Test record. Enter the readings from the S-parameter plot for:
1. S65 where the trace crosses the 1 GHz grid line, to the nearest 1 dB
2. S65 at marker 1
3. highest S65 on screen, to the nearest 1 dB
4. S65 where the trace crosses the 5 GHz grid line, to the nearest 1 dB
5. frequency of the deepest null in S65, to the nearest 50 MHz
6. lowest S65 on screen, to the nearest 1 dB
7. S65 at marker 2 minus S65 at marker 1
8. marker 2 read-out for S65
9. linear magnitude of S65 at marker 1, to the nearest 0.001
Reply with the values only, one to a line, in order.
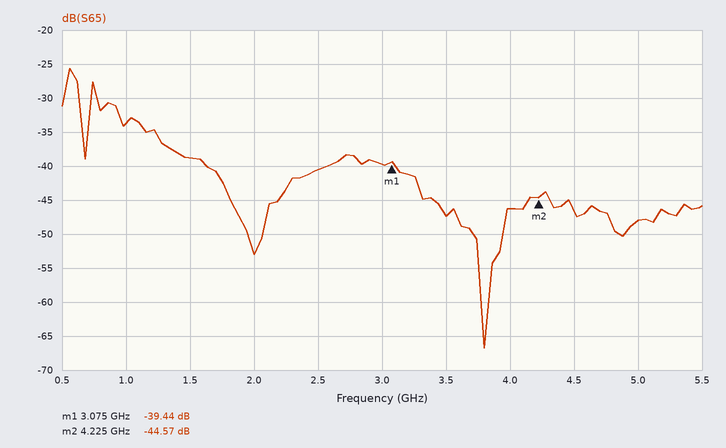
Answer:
-34 dB
-39.44 dB
-26 dB
-48 dB
3.80 GHz
-67 dB
-5.13 dB
-44.57 dB
0.011
